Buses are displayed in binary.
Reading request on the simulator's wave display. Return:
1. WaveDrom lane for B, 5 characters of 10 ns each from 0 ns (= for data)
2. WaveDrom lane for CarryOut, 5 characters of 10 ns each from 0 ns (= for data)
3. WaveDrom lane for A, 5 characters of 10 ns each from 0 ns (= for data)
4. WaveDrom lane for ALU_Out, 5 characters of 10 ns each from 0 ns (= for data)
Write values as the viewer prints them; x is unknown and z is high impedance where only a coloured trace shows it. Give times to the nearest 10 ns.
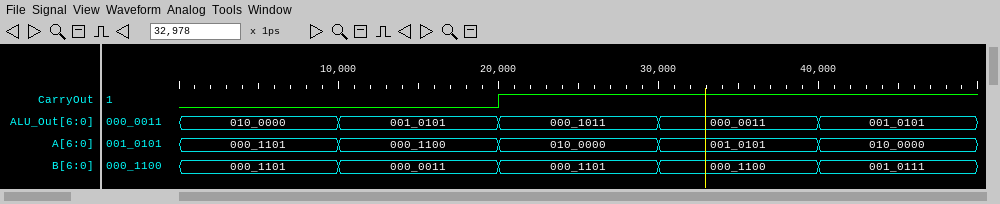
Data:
{name: 'B', wave: '=====', data: '000_1101 000_0011 000_1101 000_1100 001_0111'}
{name: 'CarryOut', wave: '0.1..'}
{name: 'A', wave: '=====', data: '000_1101 000_1100 010_0000 001_0101 010_0000'}
{name: 'ALU_Out', wave: '=====', data: '010_0000 001_0101 000_1011 000_0011 001_0101'}
